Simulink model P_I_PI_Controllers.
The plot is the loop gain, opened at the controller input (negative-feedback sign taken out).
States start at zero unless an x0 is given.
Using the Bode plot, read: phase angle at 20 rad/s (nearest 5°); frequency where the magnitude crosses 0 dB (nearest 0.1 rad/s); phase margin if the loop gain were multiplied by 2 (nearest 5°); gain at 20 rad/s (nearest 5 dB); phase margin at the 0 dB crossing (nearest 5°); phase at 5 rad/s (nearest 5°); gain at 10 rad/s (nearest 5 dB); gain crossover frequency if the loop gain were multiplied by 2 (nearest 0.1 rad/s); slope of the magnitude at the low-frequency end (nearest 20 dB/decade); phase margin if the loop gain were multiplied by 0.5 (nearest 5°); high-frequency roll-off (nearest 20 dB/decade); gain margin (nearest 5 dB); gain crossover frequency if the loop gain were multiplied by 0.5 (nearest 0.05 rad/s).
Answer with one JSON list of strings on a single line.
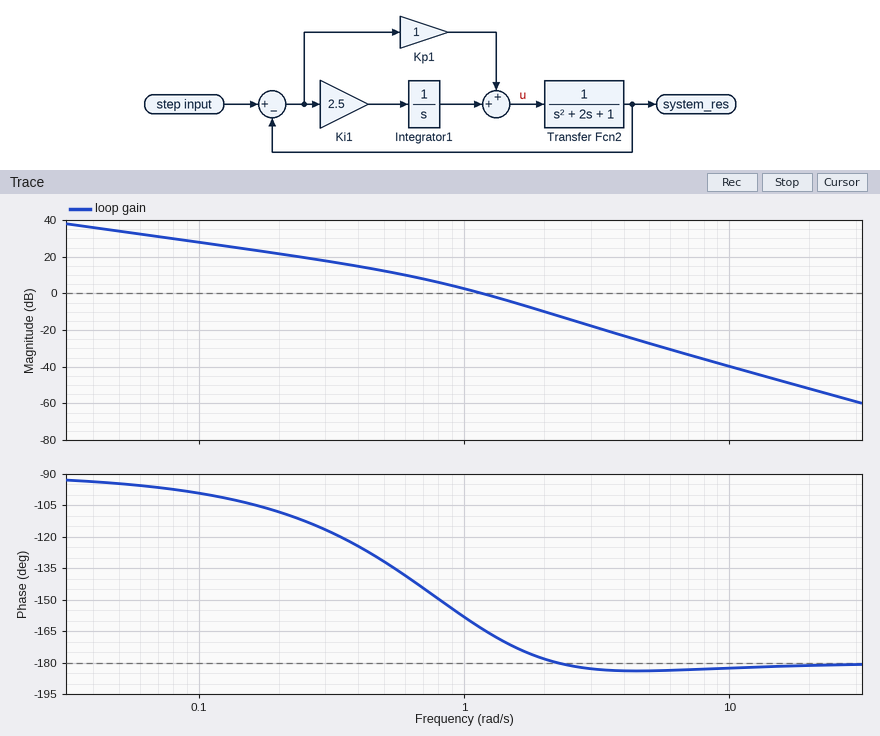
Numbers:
["-180°", "1.2 rad/s", "5°", "-50 dB", "15°", "-185°", "-40 dB", "1.6 rad/s", "-20 dB/decade", "30°", "-40 dB/decade", "10 dB", "0.80 rad/s"]
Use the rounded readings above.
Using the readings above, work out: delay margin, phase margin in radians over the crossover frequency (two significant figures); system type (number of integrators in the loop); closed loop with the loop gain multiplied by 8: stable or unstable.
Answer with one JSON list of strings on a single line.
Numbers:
["0.22 s", "1", "unstable"]
